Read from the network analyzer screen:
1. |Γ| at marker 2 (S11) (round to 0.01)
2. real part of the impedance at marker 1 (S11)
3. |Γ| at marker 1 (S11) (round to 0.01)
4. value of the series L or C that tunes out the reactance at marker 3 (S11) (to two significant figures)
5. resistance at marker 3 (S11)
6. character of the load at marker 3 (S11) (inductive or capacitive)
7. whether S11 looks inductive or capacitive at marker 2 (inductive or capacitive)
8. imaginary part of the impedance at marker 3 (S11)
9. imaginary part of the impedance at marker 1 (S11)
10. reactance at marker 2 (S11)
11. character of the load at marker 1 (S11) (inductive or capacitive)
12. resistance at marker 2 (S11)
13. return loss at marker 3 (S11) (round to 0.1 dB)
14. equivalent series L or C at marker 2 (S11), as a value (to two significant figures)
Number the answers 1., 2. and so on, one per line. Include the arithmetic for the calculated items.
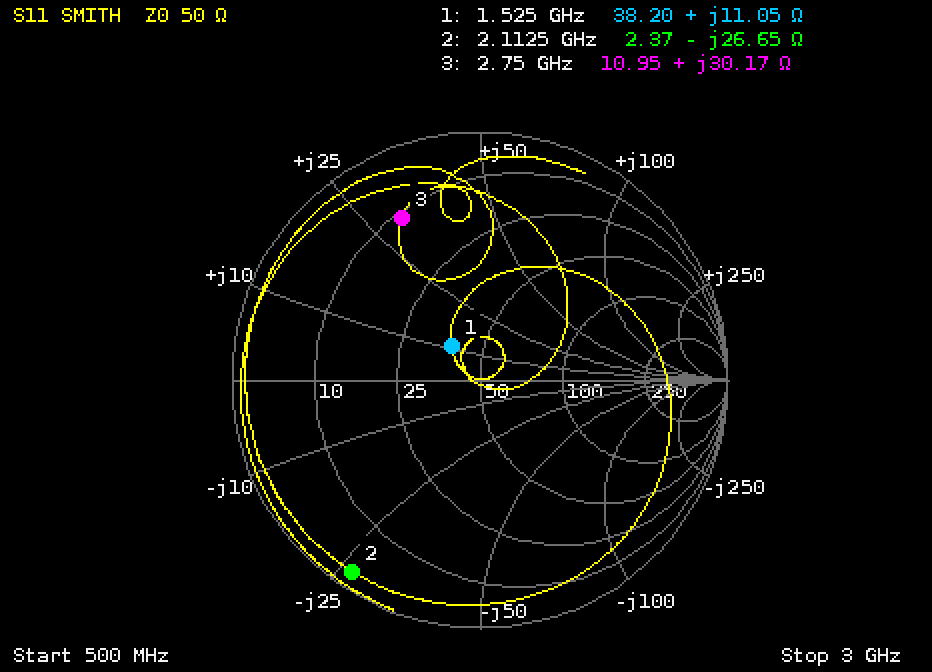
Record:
1. 0.93
2. 38.20 Ω
3. 0.18
4. C = 1/(2π × 2.75 GHz × 30.17 Ω) ≈ 1.9 pF
5. 10.95 Ω
6. inductive
7. capacitive
8. +30.17 Ω
9. +11.05 Ω
10. -26.65 Ω
11. inductive
12. 2.37 Ω
13. 2.8 dB
14. C = 1/(2π × 2.1125 GHz × 26.65 Ω) ≈ 2.8 pF
